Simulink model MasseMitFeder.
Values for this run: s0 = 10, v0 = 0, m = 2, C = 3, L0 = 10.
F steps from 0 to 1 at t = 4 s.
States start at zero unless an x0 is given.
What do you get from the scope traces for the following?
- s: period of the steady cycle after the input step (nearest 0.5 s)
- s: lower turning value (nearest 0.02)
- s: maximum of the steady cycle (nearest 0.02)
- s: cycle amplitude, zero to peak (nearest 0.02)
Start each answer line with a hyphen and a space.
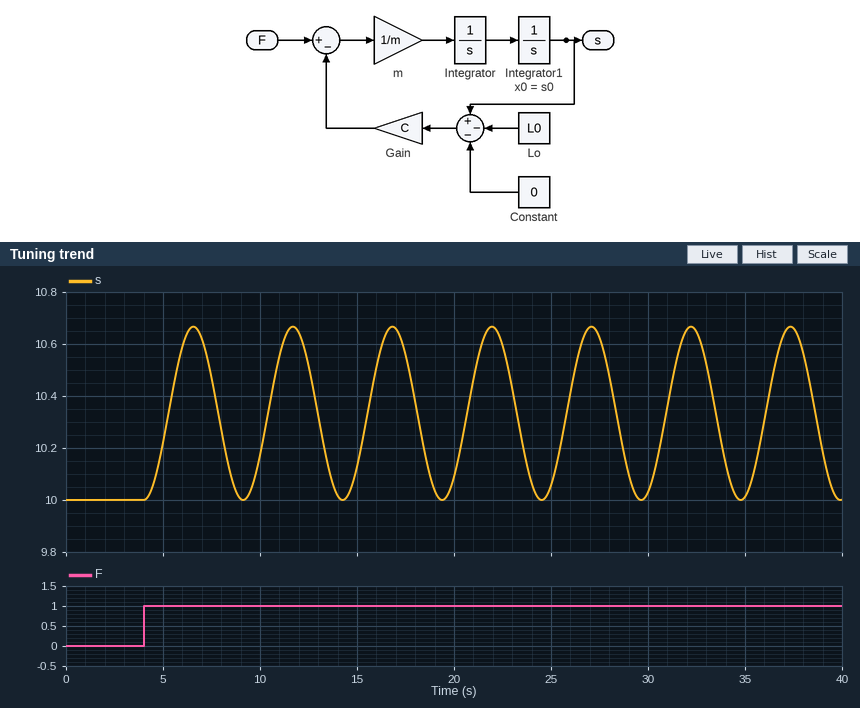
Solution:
- 5.0 s
- 10.00
- 10.66
- 0.34
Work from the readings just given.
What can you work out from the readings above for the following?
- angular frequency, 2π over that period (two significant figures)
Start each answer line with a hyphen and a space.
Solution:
- 1.3 rad/s
